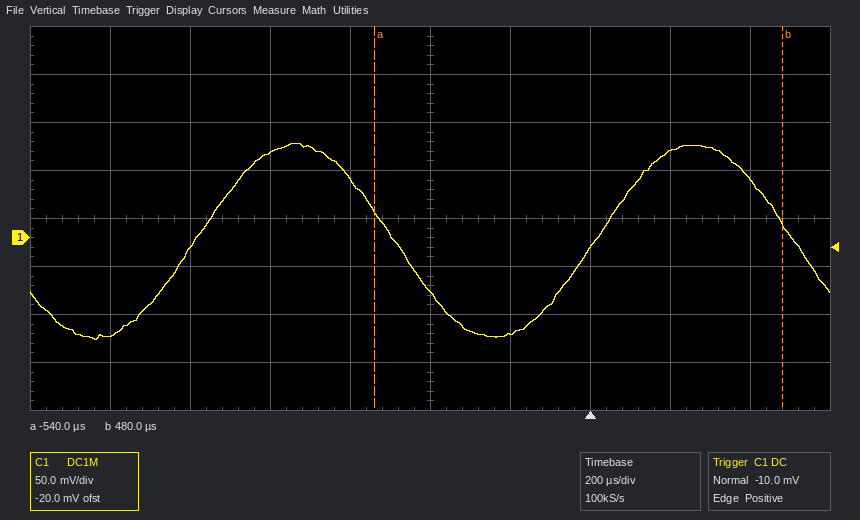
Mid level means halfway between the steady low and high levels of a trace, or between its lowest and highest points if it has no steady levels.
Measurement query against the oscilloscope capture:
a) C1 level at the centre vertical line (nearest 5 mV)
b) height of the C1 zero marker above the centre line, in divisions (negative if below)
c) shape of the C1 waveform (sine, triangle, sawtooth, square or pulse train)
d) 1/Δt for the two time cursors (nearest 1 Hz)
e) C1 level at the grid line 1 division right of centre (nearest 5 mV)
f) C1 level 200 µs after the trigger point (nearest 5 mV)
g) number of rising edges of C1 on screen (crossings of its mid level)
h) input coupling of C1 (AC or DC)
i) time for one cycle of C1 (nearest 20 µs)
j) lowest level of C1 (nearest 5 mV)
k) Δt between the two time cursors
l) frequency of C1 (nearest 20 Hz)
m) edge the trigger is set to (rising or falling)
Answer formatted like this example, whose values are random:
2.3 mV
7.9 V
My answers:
-55 mV
-0.4 div
sine
980 Hz
-100 mV
90 mV
2
DC
1.00 ms
-105 mV
1.02 ms
1.00 kHz
rising
